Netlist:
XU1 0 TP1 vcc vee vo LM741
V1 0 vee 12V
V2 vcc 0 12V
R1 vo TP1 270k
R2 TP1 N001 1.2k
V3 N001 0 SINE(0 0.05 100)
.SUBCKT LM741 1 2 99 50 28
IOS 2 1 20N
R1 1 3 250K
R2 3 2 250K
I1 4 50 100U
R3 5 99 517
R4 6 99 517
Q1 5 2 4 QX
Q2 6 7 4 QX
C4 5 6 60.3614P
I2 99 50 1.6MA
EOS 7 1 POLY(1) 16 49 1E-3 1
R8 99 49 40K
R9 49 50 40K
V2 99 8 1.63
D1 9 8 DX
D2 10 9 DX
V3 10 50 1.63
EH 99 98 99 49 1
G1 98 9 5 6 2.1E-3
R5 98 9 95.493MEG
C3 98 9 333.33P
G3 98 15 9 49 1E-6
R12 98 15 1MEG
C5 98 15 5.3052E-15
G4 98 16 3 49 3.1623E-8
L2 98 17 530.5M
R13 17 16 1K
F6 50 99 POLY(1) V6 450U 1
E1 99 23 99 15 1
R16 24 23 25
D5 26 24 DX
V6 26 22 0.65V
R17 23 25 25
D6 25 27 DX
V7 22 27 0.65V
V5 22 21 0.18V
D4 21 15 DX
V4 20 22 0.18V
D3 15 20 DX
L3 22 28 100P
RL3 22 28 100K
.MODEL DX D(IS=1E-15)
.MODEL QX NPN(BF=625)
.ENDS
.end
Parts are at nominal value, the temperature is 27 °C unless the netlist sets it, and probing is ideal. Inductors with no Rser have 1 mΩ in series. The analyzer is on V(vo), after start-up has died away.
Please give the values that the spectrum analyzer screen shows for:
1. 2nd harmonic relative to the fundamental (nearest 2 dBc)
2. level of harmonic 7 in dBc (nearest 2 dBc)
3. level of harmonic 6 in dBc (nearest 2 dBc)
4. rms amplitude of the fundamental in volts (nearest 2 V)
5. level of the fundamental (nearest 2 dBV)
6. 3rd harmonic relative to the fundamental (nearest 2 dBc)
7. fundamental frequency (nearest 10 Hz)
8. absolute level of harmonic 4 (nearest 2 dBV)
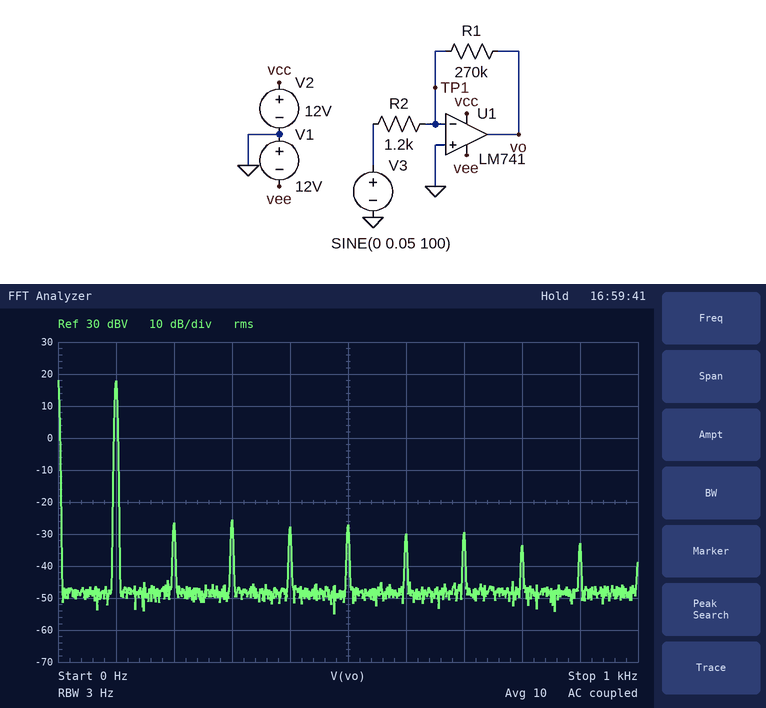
-44 dBc
-48 dBc
-48 dBc
8 V
18 dBV
-44 dBc
100 Hz
-28 dBV
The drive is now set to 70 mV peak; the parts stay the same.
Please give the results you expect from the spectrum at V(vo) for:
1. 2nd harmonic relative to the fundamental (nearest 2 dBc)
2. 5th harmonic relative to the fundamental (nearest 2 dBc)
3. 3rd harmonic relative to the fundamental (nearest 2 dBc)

-38 dBc
-32 dBc
-18 dBc
